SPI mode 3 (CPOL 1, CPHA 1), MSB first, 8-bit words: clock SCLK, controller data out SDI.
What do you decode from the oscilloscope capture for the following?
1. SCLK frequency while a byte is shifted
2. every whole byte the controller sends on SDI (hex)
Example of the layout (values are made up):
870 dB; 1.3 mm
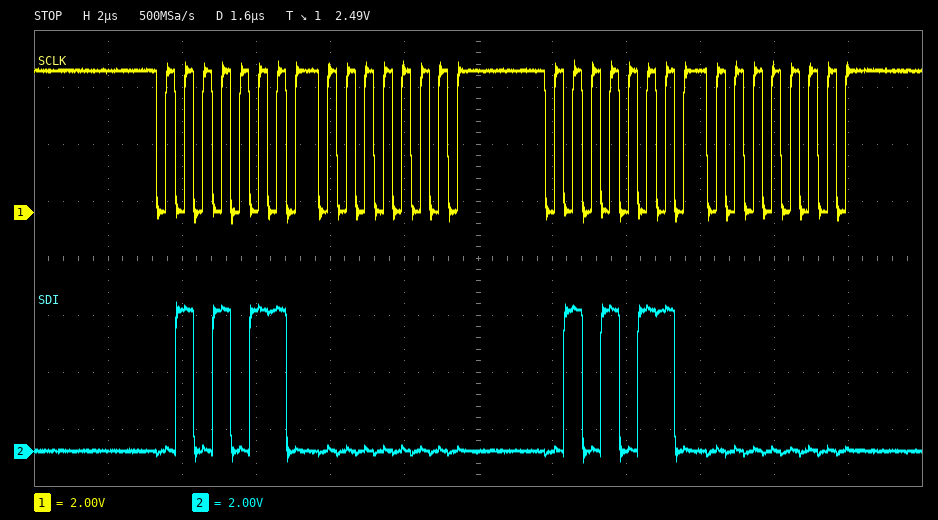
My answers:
2 MHz; 56 00 56 00
